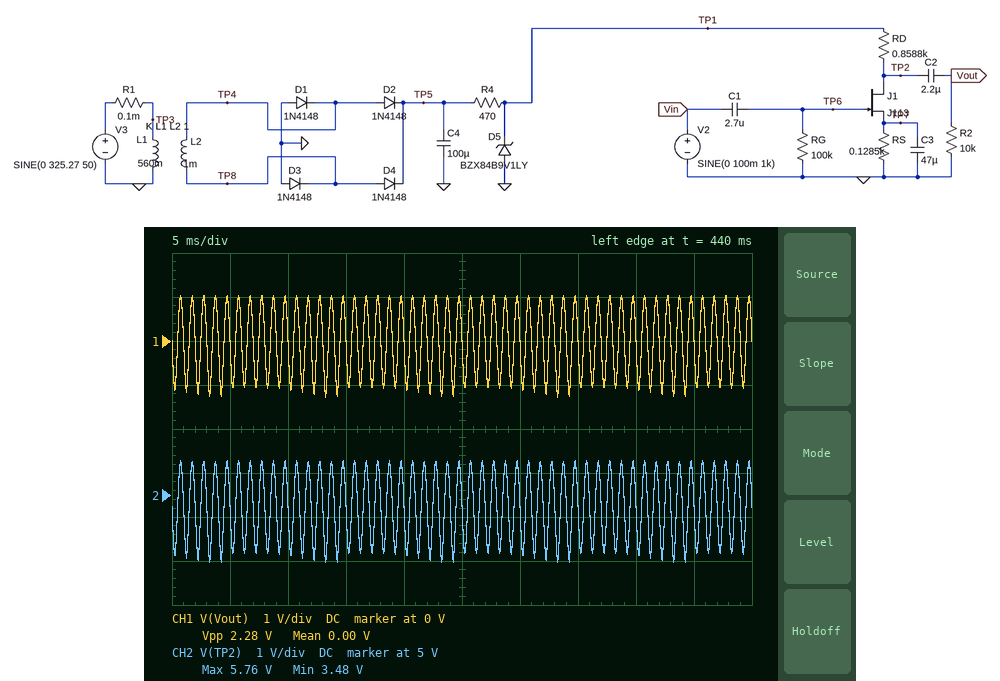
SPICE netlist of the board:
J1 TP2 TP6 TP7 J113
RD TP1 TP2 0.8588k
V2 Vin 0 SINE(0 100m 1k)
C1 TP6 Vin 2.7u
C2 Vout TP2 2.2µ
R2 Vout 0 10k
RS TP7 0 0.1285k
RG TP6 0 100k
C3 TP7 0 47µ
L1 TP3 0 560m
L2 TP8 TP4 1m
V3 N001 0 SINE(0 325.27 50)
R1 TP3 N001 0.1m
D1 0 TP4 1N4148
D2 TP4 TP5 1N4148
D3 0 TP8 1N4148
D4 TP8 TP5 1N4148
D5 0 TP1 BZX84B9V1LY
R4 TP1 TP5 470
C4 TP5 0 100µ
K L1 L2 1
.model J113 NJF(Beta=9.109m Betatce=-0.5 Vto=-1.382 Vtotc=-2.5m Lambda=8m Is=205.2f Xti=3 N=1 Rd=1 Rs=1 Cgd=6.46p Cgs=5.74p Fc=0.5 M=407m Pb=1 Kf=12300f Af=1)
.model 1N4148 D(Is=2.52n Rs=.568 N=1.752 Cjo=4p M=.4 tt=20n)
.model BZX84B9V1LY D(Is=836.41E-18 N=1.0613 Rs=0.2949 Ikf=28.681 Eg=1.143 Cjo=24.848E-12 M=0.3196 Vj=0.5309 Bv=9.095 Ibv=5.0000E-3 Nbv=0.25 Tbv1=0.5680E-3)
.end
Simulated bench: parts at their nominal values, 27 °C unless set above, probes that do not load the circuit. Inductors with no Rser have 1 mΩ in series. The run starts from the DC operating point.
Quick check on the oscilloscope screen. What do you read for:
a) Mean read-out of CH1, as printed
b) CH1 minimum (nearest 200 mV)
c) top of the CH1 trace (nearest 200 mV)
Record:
0.00 V
-1.2 V
1.0 V
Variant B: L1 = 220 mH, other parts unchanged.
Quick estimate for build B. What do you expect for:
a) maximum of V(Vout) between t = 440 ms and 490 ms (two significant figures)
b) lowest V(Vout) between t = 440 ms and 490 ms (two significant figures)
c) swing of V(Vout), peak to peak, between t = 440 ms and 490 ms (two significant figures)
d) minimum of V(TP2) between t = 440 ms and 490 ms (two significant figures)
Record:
1.0 V
-1.1 V
2.1 V
3.7 V
